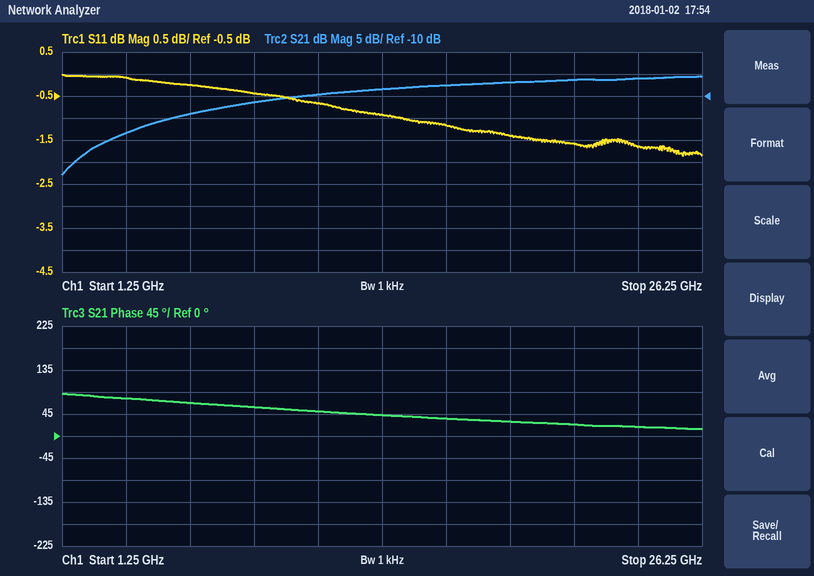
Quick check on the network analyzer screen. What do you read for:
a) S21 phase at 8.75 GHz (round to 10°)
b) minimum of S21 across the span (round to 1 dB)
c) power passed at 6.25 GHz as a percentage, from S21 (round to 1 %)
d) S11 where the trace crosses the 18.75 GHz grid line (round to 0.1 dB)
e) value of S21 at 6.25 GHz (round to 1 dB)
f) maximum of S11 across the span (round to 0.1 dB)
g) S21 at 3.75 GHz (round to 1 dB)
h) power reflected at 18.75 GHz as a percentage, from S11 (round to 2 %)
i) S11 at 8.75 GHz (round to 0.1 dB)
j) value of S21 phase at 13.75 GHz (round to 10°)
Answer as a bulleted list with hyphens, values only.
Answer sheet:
- 60°
- -28 dB
- 4 %
- -1.4 dB
- -14 dB
- 0.0 dB
- -18 dB
- 72 %
- -0.4 dB
- 40°
